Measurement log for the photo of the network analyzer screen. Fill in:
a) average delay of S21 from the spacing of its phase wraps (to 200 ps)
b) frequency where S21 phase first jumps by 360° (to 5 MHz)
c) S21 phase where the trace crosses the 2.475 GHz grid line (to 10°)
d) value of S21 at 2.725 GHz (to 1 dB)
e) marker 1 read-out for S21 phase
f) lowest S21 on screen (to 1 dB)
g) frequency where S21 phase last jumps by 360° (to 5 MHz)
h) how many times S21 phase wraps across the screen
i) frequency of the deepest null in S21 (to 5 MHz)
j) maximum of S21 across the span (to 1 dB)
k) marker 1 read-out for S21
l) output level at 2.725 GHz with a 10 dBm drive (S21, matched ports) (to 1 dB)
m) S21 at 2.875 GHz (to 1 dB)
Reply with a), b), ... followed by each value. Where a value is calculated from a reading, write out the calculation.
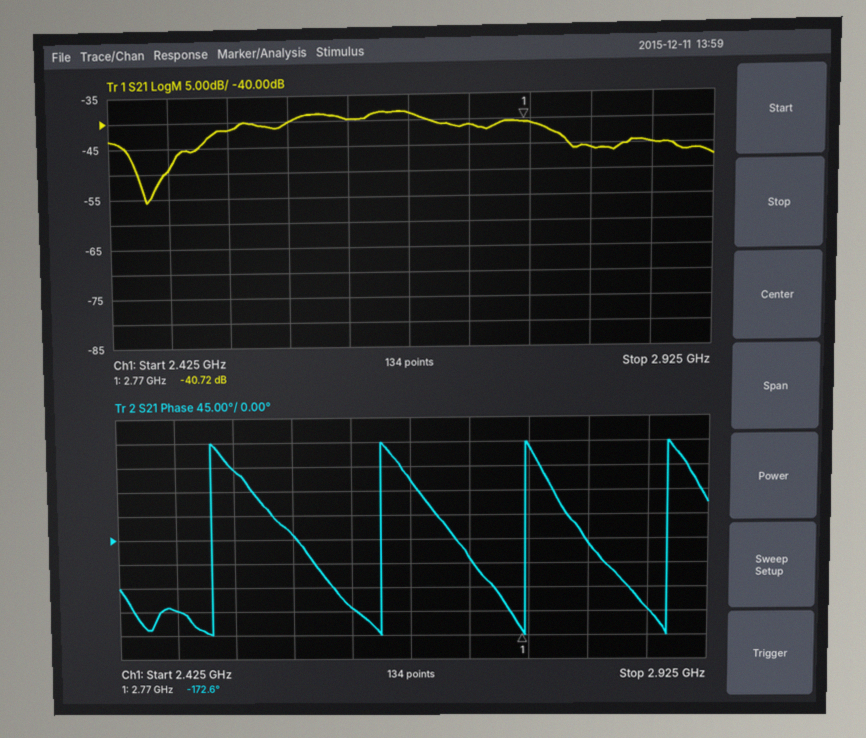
a) 3 cycles / (2.890 GHz − 2.505 GHz) ≈ 7.8 ns
b) 2.505 GHz
c) -130°
d) -41 dB
e) -172.6°
f) -56 dB
g) 2.890 GHz
h) 4
i) 2.455 GHz
j) -38 dB
k) -40.72 dB
l) 10 dBm + (-41 dB) = -31 dBm
m) -45 dB
